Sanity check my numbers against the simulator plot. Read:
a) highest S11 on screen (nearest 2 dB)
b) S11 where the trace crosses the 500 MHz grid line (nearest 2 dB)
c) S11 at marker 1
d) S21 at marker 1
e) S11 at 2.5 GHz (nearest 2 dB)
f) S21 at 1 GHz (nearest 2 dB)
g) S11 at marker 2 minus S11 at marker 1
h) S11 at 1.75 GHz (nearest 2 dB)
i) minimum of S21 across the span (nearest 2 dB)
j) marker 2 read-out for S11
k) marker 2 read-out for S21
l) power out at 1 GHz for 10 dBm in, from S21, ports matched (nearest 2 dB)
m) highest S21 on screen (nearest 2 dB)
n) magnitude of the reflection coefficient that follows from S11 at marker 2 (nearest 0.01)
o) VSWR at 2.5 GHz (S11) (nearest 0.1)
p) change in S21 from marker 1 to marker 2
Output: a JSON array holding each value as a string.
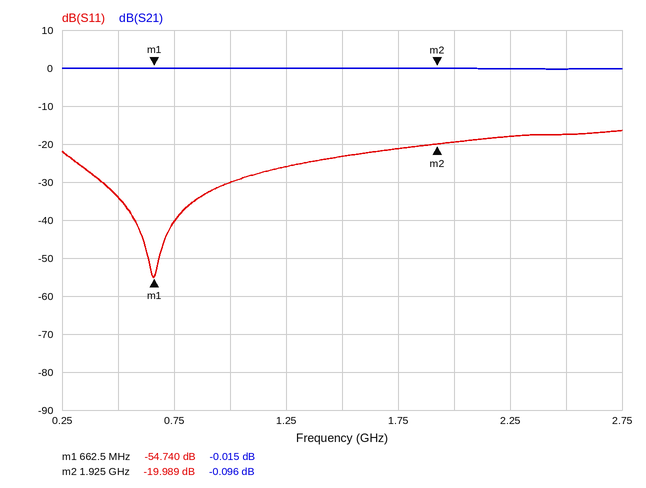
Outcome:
["-16 dB", "-34 dB", "-54.740 dB", "-0.015 dB", "-18 dB", "0 dB", "34.751 dB", "-22 dB", "0 dB", "-19.989 dB", "-0.096 dB", "10 dBm", "0 dB", "0.10", "1.3", "-0.081 dB"]
